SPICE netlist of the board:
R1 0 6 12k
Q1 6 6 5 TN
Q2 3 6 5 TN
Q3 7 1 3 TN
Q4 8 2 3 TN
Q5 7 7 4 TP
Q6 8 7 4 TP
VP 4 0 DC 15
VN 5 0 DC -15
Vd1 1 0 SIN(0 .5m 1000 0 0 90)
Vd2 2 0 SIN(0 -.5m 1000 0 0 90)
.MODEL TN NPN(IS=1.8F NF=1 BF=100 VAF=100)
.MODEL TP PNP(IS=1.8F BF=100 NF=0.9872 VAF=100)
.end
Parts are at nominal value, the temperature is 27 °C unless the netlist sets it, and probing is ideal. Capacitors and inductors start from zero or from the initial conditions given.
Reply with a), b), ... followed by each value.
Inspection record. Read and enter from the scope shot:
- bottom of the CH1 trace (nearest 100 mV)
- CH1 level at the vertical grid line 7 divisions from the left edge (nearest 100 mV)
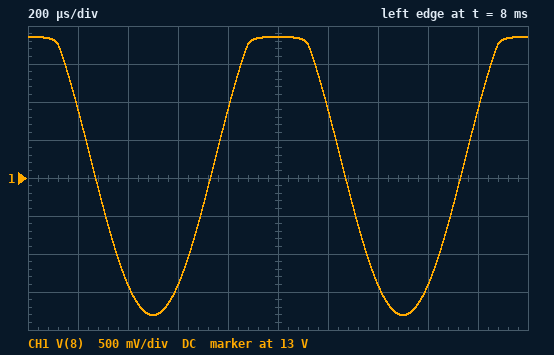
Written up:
a) 11.2 V
b) 11.6 V
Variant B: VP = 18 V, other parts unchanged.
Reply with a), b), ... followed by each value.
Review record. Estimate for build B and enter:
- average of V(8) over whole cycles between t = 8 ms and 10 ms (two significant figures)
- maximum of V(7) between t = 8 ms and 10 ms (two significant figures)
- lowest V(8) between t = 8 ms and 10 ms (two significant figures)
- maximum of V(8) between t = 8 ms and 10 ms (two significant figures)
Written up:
a) 16 V
b) 17 V
c) 14 V
d) 18 V
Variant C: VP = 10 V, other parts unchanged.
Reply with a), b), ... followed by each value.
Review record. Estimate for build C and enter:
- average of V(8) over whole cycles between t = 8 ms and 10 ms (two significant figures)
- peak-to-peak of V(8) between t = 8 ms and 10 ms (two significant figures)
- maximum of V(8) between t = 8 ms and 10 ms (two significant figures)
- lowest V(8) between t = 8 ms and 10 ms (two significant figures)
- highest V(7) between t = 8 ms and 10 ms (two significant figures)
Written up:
a) 8.2 V
b) 3.6 V
c) 9.9 V
d) 6.3 V
e) 9.3 V
